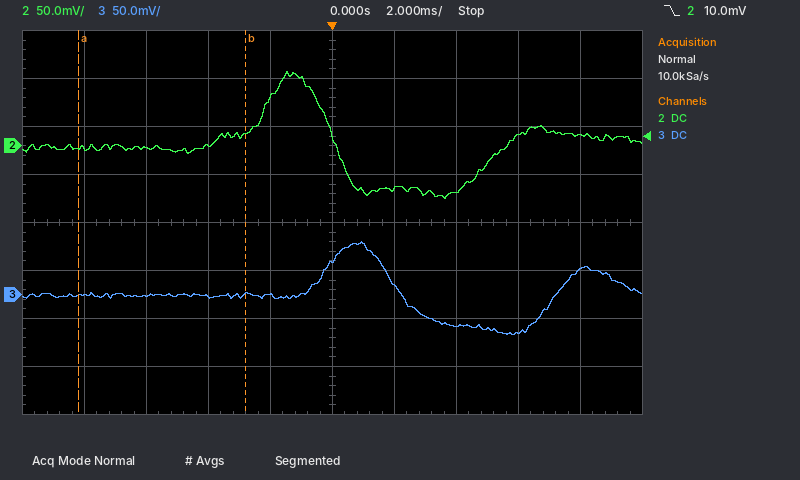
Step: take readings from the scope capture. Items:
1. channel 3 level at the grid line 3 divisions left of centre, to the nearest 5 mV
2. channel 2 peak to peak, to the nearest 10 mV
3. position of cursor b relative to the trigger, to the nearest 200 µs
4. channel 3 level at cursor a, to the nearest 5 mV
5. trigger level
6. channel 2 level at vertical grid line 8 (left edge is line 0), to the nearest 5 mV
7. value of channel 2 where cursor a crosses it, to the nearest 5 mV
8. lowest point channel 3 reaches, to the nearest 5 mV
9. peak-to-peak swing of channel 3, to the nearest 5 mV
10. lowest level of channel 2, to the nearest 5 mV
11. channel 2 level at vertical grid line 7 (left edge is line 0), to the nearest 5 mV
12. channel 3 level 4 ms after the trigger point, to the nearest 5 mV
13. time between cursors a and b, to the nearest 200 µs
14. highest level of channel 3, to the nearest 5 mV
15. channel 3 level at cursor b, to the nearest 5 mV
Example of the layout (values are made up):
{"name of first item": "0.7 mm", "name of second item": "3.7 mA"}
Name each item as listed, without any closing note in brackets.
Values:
{"channel 3 level at the grid line 3 divisions left of centre, to the nearest 5 mV": "0 mV", "channel 2 peak to peak, to the nearest 10 mV": "130 mV", "position of cursor b relative to the trigger, to the nearest 200 µs": "-2.8 ms", "channel 3 level at cursor a, to the nearest 5 mV": "0 mV", "trigger level": "10.0 mV", "channel 2 level at vertical grid line 8 (left edge is line 0), to the nearest 5 mV": "10 mV", "value of channel 2 where cursor a crosses it, to the nearest 5 mV": "0 mV", "lowest point channel 3 reaches, to the nearest 5 mV": "-40 mV", "peak-to-peak swing of channel 3, to the nearest 5 mV": "95 mV", "lowest level of channel 2, to the nearest 5 mV": "-55 mV", "channel 2 level at vertical grid line 7 (left edge is line 0), to the nearest 5 mV": "-50 mV", "channel 3 level 4 ms after the trigger point, to the nearest 5 mV": "-35 mV", "time between cursors a and b, to the nearest 200 µs": "5.4 ms", "highest level of channel 3, to the nearest 5 mV": "55 mV", "channel 3 level at cursor b, to the nearest 5 mV": "0 mV"}
